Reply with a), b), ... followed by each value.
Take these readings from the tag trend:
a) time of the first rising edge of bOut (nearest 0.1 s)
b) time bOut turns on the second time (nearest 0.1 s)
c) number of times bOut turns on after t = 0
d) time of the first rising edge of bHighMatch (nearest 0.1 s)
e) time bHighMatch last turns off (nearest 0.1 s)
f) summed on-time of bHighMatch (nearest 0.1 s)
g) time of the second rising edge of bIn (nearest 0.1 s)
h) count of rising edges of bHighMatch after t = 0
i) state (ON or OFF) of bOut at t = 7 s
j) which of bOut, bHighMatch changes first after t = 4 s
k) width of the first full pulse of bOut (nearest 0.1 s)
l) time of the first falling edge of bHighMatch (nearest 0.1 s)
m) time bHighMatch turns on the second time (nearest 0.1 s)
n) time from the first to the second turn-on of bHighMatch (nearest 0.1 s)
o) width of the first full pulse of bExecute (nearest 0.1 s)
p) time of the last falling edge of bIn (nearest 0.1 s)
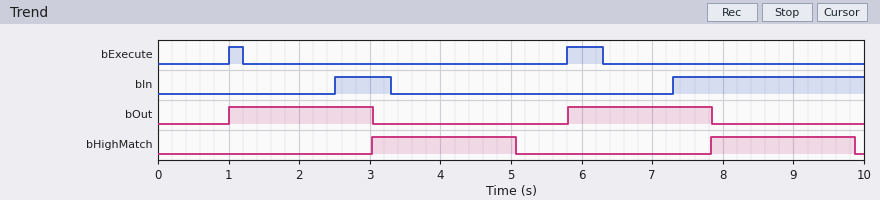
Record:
a) 1.0 s
b) 5.8 s
c) 2
d) 3.0 s
e) 9.9 s
f) 4.1 s
g) 7.3 s
h) 2
i) ON
j) bHighMatch
k) 2.0 s
l) 5.1 s
m) 7.8 s
n) 4.8 s
o) 0.2 s
p) 3.3 s
